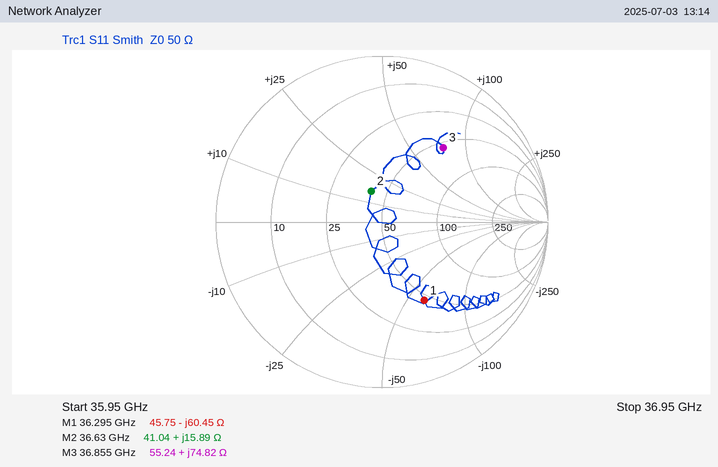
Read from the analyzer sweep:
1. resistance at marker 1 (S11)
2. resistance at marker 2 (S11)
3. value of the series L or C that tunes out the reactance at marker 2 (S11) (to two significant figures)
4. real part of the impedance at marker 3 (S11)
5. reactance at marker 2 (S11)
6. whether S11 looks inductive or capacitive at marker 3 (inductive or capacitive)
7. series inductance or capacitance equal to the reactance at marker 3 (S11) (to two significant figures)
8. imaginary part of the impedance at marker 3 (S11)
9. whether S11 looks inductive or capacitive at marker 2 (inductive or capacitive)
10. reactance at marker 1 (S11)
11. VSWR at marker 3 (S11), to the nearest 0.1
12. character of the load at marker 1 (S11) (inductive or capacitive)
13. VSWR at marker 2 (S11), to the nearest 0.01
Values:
45.75 Ω
41.04 Ω
270 fF
55.24 Ω
+15.89 Ω
inductive
320 pH
+74.82 Ω
inductive
-60.45 Ω
3.8
capacitive
1.49
